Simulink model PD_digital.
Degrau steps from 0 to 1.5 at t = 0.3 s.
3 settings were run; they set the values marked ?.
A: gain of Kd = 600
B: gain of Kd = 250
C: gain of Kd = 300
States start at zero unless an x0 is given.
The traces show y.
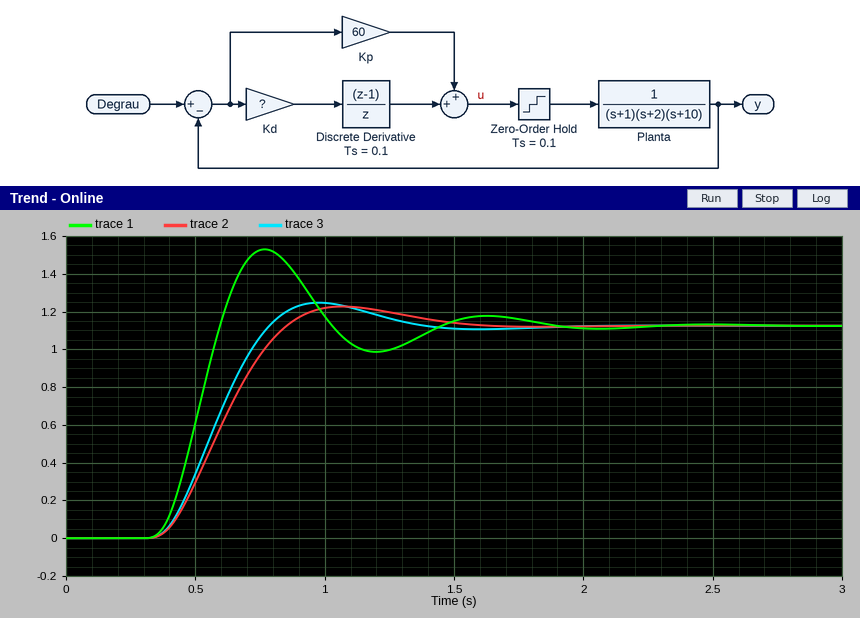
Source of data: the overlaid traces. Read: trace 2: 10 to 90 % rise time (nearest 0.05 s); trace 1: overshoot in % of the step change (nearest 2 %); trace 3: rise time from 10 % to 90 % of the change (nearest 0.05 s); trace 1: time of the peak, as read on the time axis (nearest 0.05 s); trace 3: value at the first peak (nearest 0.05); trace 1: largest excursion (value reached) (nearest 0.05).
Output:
0.35 s
36 %
0.30 s
0.75 s
1.25
1.55
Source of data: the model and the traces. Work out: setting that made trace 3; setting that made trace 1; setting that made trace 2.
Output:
C
A
B
